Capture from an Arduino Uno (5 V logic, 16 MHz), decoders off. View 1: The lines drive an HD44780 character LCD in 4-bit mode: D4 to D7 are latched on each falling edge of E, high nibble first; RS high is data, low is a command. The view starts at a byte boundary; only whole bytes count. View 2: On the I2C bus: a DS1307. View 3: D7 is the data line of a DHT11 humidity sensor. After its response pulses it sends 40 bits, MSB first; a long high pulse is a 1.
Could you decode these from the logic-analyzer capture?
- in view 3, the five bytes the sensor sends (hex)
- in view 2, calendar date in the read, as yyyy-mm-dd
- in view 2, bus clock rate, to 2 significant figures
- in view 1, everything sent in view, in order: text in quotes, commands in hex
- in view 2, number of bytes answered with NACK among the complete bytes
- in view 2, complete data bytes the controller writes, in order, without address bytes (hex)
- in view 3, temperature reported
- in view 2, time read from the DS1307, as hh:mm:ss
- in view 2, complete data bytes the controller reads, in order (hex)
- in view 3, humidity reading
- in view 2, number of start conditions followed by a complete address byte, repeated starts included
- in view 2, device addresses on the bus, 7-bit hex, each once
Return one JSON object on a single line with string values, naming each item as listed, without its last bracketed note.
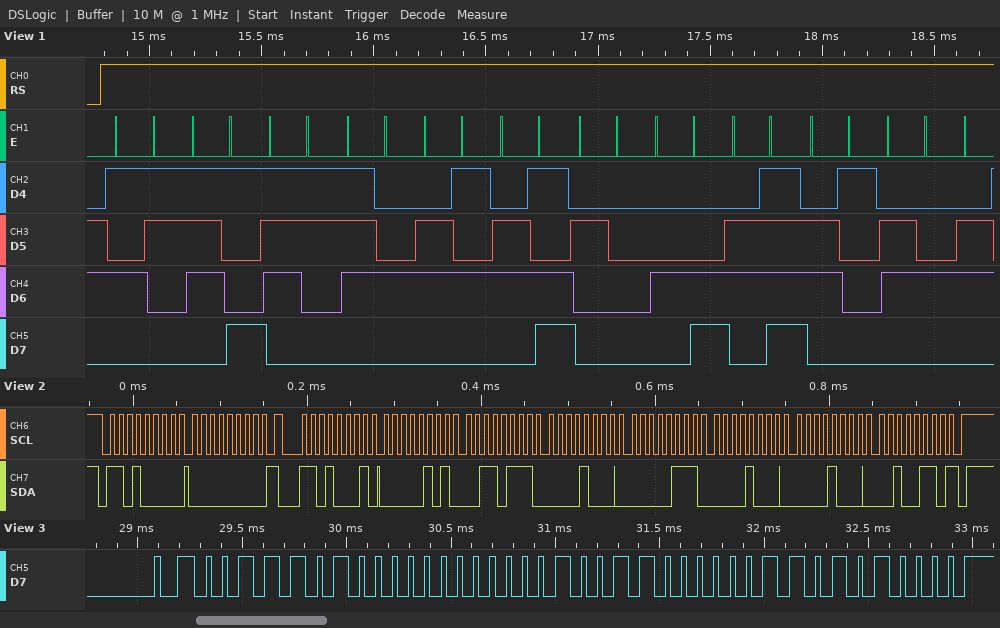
{"in view 3, the five bytes the sensor sends": "3A 00 13 03 50", "in view 2, calendar date in the read, as yyyy-mm-dd": "2026-08-08", "in view 2, bus clock rate, to 2 significant figures": "100 kHz", "in view 1, everything sent in view, in order: text in quotes, commands in hex": "\"System Load\"", "in view 2, number of bytes answered with NACK among the complete bytes": "1", "in view 2, complete data bytes the controller writes, in order, without address bytes": "00", "in view 3, temperature reported": "19.3 °C", "in view 2, time read from the DS1307, as hh:mm:ss": "08:37:05", "in view 2, complete data bytes the controller reads, in order": "05 37 08 07 08 08 26", "in view 3, humidity reading": "58 %", "in view 2, number of start conditions followed by a complete address byte, repeated starts included": "2", "in view 2, device addresses on the bus, 7-bit hex, each once": "0x68"}
